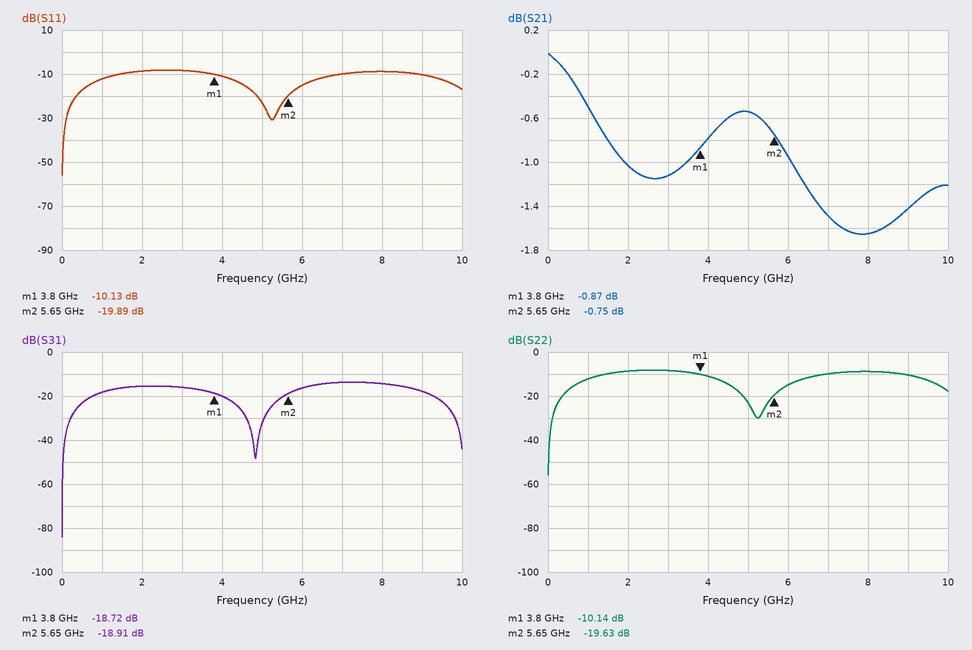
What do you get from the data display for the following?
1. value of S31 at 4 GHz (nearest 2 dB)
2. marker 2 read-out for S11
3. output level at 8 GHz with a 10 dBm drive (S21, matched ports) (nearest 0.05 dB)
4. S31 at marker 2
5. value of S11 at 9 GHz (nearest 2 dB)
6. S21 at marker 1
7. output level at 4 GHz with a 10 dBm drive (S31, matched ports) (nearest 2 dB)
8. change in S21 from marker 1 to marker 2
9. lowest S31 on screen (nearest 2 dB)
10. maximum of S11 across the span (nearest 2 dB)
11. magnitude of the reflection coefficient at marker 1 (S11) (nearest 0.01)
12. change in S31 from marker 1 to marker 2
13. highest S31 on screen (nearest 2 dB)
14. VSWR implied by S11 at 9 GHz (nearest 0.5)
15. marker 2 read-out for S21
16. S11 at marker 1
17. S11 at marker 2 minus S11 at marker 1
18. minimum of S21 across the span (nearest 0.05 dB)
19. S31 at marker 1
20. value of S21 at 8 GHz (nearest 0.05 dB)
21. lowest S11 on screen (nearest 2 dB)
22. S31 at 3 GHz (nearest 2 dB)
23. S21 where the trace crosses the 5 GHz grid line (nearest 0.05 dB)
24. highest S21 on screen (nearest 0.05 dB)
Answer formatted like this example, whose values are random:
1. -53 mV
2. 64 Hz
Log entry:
1. -20 dB
2. -19.89 dB
3. 8.35 dBm
4. -18.91 dB
5. -10 dB
6. -0.87 dB
7. -10 dBm
8. 0.12 dB
9. -84 dB
10. -8 dB
11. 0.31
12. -0.19 dB
13. -14 dB
14. 2.0
15. -0.75 dB
16. -10.13 dB
17. -9.76 dB
18. -1.65 dB
19. -18.72 dB
20. -1.65 dB
21. -56 dB
22. -16 dB
23. -0.55 dB
24. 0.00 dB
